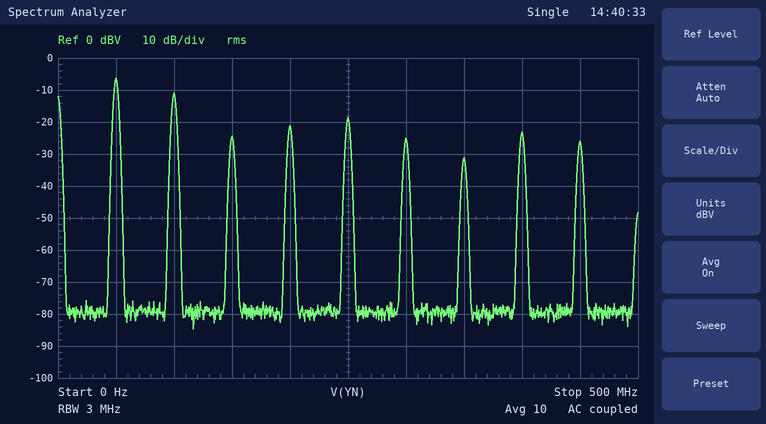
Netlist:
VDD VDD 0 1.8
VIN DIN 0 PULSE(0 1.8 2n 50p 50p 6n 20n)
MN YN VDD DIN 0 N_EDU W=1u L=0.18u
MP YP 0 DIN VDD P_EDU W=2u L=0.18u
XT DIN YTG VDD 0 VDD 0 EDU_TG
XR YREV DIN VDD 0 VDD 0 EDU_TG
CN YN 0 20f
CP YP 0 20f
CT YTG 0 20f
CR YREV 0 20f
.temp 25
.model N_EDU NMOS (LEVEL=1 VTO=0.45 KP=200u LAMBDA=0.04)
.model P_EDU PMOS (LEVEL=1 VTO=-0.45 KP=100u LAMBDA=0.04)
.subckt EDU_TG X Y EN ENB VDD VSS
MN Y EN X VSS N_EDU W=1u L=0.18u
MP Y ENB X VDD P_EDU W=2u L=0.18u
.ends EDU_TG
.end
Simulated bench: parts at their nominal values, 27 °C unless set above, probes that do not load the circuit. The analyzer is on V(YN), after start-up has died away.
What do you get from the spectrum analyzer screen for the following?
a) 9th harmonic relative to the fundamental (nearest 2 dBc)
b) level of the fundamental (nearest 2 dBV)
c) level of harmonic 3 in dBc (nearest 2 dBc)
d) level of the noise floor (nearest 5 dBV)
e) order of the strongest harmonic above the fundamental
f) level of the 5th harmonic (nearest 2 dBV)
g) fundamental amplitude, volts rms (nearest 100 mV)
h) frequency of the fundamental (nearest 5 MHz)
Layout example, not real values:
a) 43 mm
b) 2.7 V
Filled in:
a) -20 dBc
b) -6 dBV
c) -18 dBc
d) -80 dBV
e) 2
f) -18 dBV
g) 500 mV
h) 50 MHz
